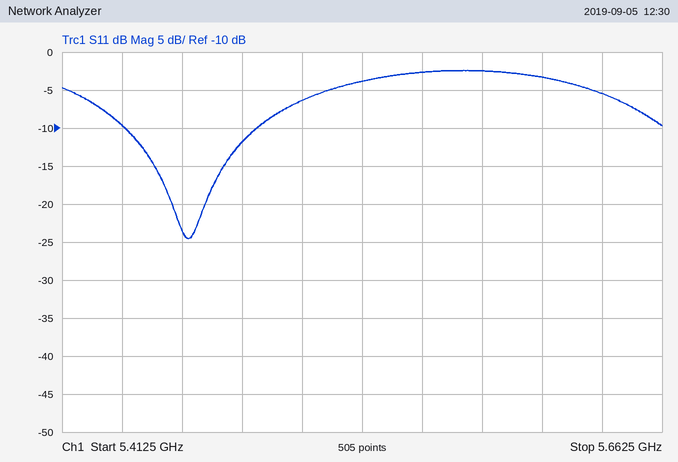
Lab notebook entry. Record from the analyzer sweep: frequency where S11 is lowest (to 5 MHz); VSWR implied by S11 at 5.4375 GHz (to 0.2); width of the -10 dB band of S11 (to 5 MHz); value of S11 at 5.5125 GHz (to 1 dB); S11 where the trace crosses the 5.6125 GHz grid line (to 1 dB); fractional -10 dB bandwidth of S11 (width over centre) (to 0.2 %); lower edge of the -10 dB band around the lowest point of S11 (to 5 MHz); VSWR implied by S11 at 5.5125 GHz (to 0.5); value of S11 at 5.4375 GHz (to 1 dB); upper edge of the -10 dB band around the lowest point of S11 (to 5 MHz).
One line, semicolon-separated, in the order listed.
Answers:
5.465 GHz; 2.0; 55 MHz; -6 dB; -3 dB; 1.0 %; 5.440 GHz; 3.0; -10 dB; 5.495 GHz
